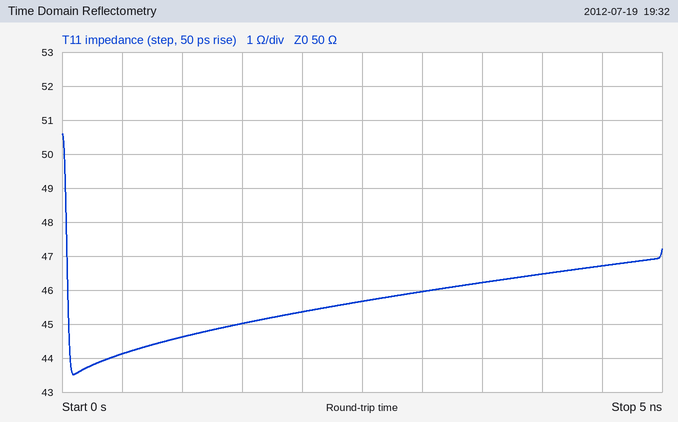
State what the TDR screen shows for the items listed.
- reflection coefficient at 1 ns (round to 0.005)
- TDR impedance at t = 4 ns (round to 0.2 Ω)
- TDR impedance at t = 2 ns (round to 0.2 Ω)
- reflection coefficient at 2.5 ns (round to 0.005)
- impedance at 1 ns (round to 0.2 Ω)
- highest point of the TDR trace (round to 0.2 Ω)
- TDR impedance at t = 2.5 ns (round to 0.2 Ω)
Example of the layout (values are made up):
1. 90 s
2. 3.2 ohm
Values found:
1. -0.055
2. 46.4 Ω
3. 45.4 Ω
4. -0.045
5. 44.6 Ω
6. 50.6 Ω
7. 45.6 Ω
